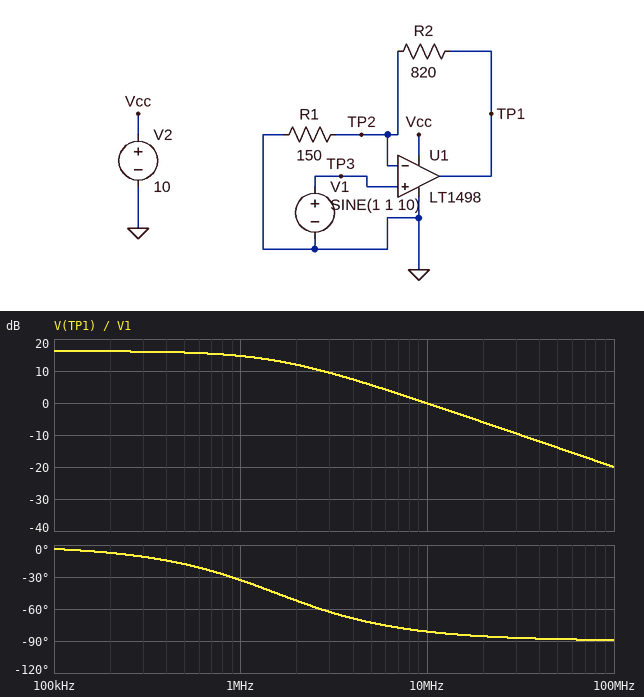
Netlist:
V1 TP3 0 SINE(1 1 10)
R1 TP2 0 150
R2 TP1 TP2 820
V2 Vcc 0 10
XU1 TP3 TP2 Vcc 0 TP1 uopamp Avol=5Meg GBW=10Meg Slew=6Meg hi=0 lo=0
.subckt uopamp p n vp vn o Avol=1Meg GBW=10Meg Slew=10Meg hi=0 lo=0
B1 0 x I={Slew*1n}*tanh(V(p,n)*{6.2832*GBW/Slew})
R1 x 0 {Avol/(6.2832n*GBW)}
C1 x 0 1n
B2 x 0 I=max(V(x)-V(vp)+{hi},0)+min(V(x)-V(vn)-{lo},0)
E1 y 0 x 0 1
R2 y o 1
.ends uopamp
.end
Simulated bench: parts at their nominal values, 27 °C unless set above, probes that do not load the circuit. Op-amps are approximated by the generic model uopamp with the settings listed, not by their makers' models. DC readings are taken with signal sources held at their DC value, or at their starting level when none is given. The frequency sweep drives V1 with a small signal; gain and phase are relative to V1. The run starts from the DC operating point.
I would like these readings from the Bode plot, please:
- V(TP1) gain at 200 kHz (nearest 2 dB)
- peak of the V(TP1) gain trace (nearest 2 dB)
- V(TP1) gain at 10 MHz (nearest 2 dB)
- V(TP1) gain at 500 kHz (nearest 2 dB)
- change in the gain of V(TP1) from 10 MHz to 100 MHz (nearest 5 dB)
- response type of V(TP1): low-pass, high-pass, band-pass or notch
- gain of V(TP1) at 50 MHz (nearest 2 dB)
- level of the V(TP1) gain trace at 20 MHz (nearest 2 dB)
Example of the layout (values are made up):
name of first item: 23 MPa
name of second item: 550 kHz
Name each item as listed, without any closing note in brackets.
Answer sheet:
V(TP1) gain at 200 kHz: 16 dB
peak of the V(TP1) gain trace: 16 dB
V(TP1) gain at 10 MHz: 0 dB
V(TP1) gain at 500 kHz: 16 dB
change in the gain of V(TP1) from 10 MHz to 100 MHz: -20 dB
response type of V(TP1): low-pass, high-pass, band-pass or notch: low-pass
gain of V(TP1) at 50 MHz: -14 dB
level of the V(TP1) gain trace at 20 MHz: -6 dB
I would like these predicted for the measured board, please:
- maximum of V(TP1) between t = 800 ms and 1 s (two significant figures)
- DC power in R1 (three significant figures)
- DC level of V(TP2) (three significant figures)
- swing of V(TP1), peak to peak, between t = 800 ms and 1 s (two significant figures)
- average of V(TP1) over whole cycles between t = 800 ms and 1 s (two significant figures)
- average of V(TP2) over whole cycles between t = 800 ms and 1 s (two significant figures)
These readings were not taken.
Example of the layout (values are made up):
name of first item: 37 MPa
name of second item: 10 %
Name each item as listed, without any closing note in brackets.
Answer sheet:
maximum of V(TP1) between t = 800 ms and 1 s: 10 V
DC power in R1: 6.67 mW
DC level of V(TP2): 1.00 V
swing of V(TP1), peak to peak, between t = 800 ms and 1 s: 10 V
average of V(TP1) over whole cycles between t = 800 ms and 1 s: 5.9 V
average of V(TP2) over whole cycles between t = 800 ms and 1 s: 910 mV
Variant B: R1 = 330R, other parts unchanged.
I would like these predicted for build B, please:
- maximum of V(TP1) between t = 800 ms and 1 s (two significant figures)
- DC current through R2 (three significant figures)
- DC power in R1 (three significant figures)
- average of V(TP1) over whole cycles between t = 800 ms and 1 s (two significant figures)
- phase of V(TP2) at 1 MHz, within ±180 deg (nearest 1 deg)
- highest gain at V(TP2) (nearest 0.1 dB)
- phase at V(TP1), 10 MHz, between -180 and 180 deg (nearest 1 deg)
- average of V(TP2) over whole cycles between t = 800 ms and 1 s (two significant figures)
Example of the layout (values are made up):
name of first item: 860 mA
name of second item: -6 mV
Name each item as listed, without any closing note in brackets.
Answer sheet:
maximum of V(TP1) between t = 800 ms and 1 s: 7.0 V
DC current through R2: 3.03 mA
DC power in R1: 3.03 mW
average of V(TP1) over whole cycles between t = 800 ms and 1 s: 3.5 V
phase of V(TP2) at 1 MHz, within ±180 deg: -19 deg
highest gain at V(TP2): 0 dB
phase at V(TP1), 10 MHz, between -180 and 180 deg: -74 deg
average of V(TP2) over whole cycles between t = 800 ms and 1 s: 1.0 V
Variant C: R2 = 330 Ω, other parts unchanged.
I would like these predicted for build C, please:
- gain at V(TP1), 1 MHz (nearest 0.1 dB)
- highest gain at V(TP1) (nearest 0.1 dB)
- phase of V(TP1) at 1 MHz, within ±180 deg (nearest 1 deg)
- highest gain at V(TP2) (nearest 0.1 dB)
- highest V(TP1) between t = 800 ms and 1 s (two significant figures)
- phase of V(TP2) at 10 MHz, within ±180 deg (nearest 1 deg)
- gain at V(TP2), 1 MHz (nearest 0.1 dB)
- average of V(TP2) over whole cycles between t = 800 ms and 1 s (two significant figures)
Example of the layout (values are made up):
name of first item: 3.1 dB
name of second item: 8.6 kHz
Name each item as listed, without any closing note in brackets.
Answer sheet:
gain at V(TP1), 1 MHz: 9.7 dB
highest gain at V(TP1): 10.1 dB
phase of V(TP1) at 1 MHz, within ±180 deg: -18 deg
highest gain at V(TP2): 0 dB
highest V(TP1) between t = 800 ms and 1 s: 6.4 V
phase of V(TP2) at 10 MHz, within ±180 deg: -73 deg
gain at V(TP2), 1 MHz: -0.4 dB
average of V(TP2) over whole cycles between t = 800 ms and 1 s: 1.0 V
